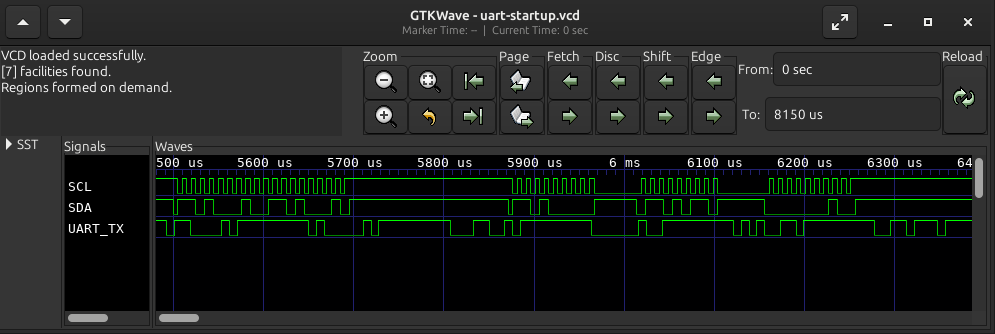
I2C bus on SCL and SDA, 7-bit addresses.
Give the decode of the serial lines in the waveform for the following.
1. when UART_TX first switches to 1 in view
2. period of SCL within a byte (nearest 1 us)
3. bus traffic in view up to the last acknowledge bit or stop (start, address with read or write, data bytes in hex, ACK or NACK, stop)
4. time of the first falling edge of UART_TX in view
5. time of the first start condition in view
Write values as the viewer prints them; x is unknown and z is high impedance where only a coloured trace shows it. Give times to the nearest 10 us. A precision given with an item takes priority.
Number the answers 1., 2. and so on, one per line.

1. 5500 us
2. 10 us
3. start, address 68 read ACK, 68 NACK, stop, start, address 68 write ACK, 6B ACK, 01 ACK, stop
4. 5490 us
5. 5500 us
